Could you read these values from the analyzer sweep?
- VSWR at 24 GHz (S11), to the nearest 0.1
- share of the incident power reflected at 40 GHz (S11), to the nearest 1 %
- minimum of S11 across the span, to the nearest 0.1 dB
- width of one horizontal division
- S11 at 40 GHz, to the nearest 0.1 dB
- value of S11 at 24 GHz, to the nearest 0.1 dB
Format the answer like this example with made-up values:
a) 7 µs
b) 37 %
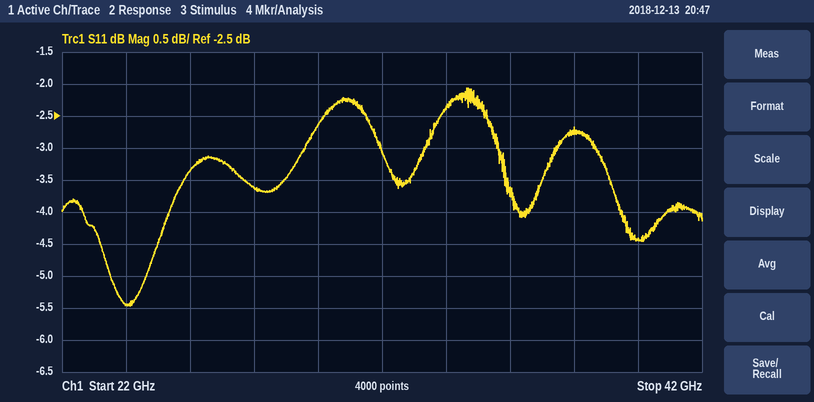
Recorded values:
a) 3.3
b) 36 %
c) -5.5 dB
d) 2 GHz
e) -4.4 dB
f) -5.4 dB
